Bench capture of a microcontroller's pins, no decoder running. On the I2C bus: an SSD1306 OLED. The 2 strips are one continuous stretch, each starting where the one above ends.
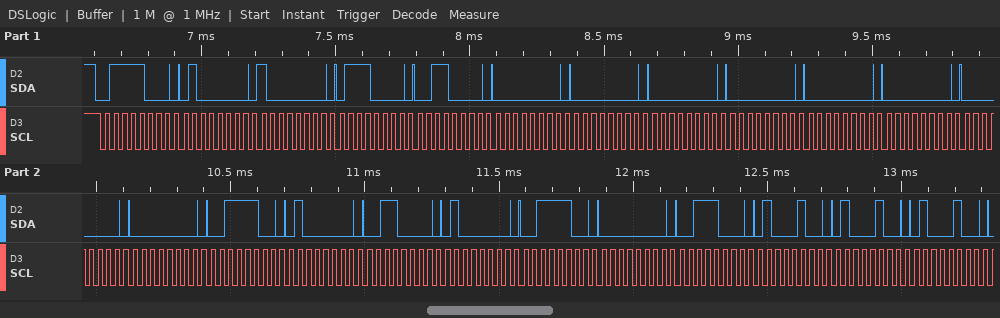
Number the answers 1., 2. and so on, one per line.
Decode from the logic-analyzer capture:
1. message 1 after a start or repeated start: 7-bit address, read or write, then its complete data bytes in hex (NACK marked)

1. 0x3C write: 40 80 70 30 00 00 00 00 00 00 00 00 3C 40 30 40 3C 00 38 44 44 44
